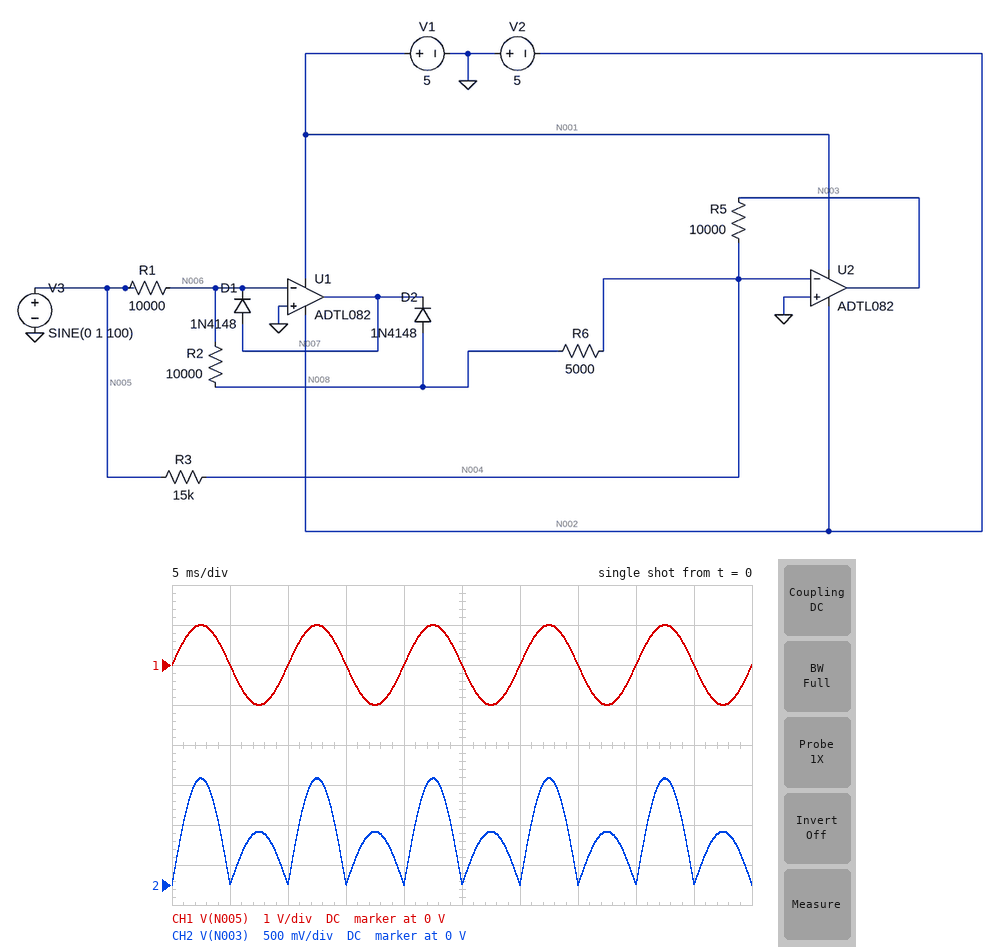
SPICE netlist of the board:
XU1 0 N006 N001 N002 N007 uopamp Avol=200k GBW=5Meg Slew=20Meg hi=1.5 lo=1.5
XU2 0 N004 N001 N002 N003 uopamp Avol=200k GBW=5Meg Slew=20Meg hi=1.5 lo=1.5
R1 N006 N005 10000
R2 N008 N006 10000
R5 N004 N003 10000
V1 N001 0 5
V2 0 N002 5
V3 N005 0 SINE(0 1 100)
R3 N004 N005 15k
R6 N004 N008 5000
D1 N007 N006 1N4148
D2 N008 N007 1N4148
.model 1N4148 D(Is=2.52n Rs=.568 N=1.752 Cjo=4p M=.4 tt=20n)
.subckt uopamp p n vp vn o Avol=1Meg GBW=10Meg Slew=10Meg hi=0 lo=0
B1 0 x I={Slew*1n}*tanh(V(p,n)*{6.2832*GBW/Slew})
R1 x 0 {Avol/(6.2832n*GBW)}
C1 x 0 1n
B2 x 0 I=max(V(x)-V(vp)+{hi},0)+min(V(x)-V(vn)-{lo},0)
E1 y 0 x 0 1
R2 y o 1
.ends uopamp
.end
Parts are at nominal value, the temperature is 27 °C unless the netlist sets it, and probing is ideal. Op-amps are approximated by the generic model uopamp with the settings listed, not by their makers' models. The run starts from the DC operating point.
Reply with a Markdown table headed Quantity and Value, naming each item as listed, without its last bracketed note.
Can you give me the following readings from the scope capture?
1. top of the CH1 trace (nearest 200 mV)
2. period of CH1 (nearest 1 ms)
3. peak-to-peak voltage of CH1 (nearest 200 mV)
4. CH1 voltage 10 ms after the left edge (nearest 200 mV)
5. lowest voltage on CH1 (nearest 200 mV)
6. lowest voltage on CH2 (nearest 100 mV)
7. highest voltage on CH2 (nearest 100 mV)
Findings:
| Quantity | Value |
|---|---|
| top of the CH1 trace | 1.0 V |
| period of CH1 | 10 ms |
| peak-to-peak voltage of CH1 | 2.0 V |
| CH1 voltage 10 ms after the left edge | 0 V |
| lowest voltage on CH1 | -1.0 V |
| lowest voltage on CH2 | 0 V |
| highest voltage on CH2 | 1.3 V |
